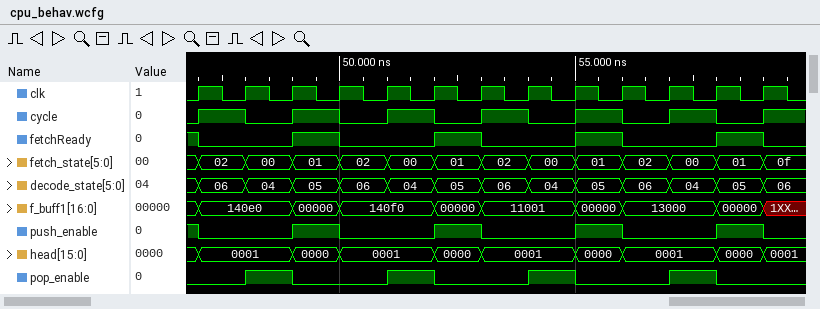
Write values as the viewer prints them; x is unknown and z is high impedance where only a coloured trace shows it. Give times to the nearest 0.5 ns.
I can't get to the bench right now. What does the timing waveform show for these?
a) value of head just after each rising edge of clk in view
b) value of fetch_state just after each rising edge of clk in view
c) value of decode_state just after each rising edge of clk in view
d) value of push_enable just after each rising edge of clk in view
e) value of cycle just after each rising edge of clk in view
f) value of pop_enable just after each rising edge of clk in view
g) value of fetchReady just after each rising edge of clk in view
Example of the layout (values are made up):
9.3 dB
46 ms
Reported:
0001, 0001, 0000, 0001, 0001, 0000, 0001, 0001, 0000, 0001, 0001, 0000, 0001
02, 00, 01, 02, 00, 01, 02, 00, 01, 02, 00, 01, 0f
06, 04, 05, 06, 04, 05, 06, 04, 05, 06, 04, 05, 06
0 0 1 0 0 1 0 0 1 0 0 1 0
1 0 1 0 1 0 1 0 1 0 1 0 1
0 1 0 0 1 0 0 1 0 0 1 0 0
0 0 1 0 0 1 0 0 1 0 0 1 0
